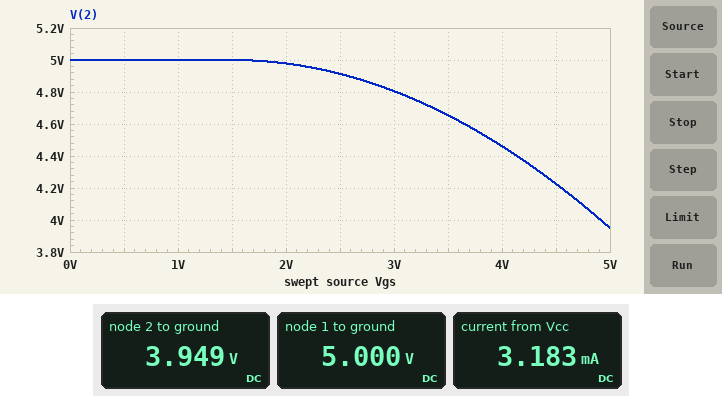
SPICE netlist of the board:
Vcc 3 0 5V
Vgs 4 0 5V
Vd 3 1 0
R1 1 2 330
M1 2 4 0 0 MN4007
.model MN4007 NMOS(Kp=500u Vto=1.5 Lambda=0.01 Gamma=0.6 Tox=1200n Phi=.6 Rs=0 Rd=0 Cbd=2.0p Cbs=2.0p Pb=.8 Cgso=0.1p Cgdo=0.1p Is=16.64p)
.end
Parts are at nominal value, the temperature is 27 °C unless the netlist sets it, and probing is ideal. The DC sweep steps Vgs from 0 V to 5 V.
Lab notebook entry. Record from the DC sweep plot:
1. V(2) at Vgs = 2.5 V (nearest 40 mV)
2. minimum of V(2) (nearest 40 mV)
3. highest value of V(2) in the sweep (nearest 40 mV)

4.92 V
3.96 V
5.00 V
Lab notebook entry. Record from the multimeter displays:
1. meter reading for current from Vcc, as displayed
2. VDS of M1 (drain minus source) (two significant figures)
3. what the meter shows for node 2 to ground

3.183 mA
3.9 V
3.949 V
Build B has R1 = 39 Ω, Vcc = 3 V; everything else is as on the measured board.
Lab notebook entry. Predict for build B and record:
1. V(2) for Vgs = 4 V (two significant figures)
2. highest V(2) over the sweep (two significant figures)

2.9 V
3.0 V
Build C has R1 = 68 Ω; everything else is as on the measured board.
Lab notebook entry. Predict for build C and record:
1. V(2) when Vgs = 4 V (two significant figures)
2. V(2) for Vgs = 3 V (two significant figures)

4.9 V
5.0 V
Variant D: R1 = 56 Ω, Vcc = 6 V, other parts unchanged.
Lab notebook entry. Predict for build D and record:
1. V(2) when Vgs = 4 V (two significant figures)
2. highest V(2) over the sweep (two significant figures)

5.9 V
6.0 V
